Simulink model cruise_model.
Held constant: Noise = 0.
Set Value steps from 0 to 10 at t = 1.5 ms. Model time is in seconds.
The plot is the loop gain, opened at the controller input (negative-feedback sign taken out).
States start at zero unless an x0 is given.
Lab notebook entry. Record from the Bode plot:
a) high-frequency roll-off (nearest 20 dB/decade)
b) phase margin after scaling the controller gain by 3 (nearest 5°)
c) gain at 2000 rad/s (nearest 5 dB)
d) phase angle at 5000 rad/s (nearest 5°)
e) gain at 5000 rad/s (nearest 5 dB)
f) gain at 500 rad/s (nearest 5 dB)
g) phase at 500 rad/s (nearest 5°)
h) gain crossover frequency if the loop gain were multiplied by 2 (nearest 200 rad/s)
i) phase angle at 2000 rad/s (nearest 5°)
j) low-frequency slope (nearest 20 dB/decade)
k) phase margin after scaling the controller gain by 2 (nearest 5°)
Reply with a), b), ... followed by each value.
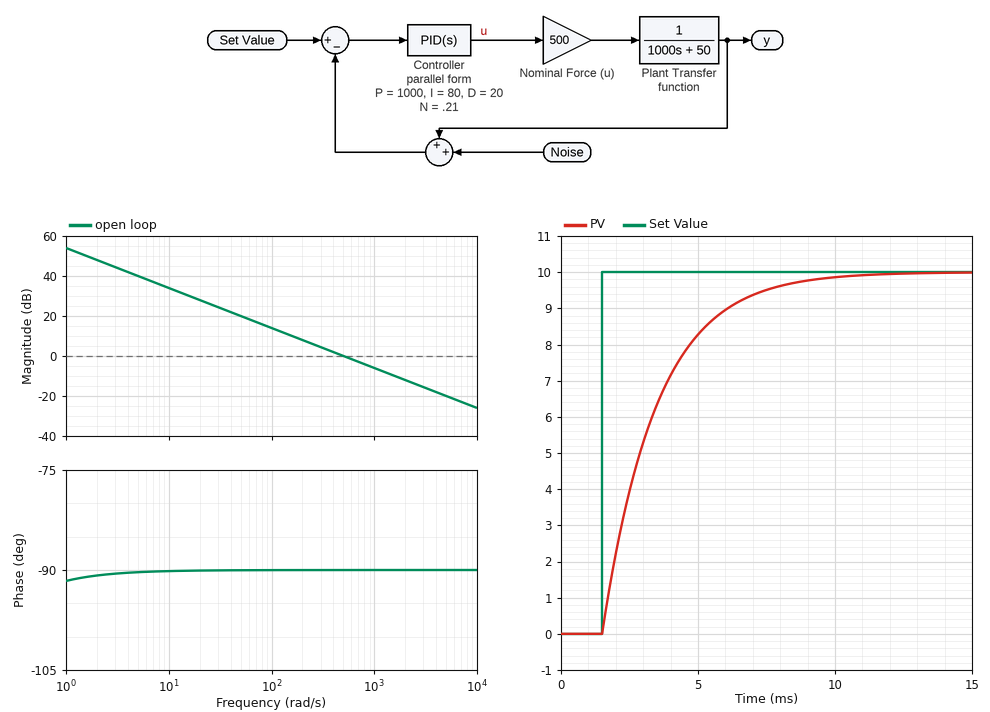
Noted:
a) -20 dB/decade
b) 90°
c) -10 dB
d) -90°
e) -20 dB
f) 0 dB
g) -90°
h) 1000 rad/s
i) -90°
j) -20 dB/decade
k) 90°
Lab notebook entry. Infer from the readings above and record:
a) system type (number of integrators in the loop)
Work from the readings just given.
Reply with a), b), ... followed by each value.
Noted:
a) 1
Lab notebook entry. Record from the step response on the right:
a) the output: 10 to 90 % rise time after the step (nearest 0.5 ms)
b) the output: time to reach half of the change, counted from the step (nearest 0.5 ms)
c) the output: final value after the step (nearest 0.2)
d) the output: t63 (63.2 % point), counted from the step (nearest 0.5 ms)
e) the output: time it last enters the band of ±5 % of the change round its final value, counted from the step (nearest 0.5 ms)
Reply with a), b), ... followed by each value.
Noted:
a) 4.5 ms
b) 1.5 ms
c) 10.0
d) 2.0 ms
e) 6.0 ms
